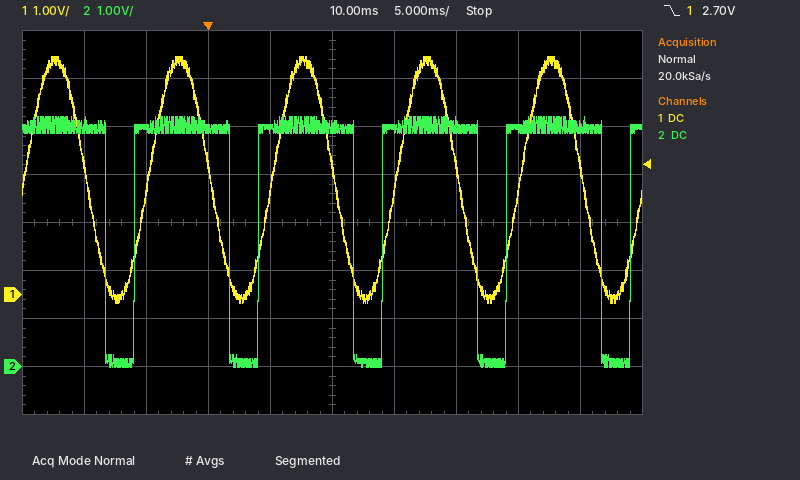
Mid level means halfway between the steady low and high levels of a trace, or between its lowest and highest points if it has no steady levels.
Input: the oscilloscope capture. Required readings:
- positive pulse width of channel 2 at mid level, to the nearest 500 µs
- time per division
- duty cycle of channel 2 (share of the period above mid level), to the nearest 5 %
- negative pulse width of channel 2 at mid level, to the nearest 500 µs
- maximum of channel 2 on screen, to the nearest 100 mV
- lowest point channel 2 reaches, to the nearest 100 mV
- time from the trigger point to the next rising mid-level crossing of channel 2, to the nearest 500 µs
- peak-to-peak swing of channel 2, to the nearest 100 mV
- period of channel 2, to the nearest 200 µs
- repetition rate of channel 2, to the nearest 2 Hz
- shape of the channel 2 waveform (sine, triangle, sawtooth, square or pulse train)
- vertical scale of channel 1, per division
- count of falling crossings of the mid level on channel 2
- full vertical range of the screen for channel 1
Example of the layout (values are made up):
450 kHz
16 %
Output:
7.5 ms
5 ms
75 %
2.5 ms
5.2 V
0.0 V
4.0 ms
5.2 V
10.0 ms
100 Hz
pulse train
1 V
5
8 V
